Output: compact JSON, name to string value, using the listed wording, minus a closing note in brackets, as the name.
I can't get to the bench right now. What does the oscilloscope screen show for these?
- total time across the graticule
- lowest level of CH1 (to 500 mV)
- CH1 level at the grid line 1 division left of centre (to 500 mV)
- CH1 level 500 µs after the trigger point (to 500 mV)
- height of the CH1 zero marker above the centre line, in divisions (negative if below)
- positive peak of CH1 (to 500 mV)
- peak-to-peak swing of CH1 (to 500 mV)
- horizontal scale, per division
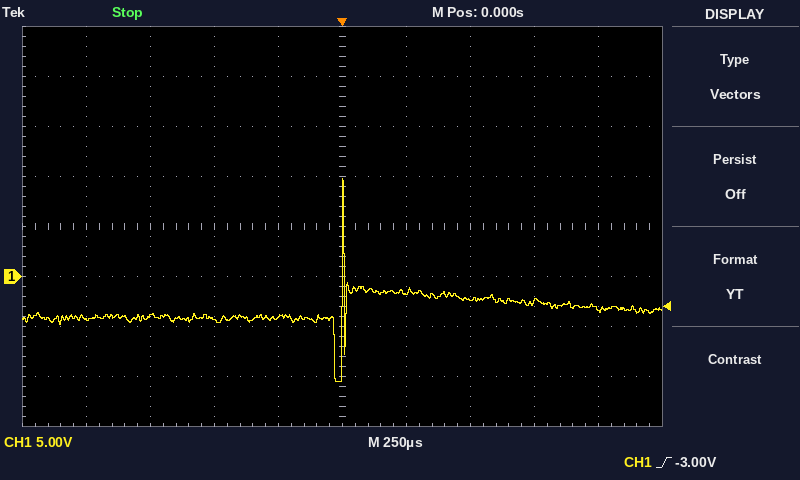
{"total time across the graticule": "2.5 ms", "lowest level of CH1": "-10.5 V", "CH1 level at the grid line 1 division left of centre": "-4.0 V", "CH1 level 500 µs after the trigger point": "-2.5 V", "height of the CH1 zero marker above the centre line, in divisions": "-1.0 div", "positive peak of CH1": "10.0 V", "peak-to-peak swing of CH1": "20.5 V", "horizontal scale, per division": "250 µs"}
